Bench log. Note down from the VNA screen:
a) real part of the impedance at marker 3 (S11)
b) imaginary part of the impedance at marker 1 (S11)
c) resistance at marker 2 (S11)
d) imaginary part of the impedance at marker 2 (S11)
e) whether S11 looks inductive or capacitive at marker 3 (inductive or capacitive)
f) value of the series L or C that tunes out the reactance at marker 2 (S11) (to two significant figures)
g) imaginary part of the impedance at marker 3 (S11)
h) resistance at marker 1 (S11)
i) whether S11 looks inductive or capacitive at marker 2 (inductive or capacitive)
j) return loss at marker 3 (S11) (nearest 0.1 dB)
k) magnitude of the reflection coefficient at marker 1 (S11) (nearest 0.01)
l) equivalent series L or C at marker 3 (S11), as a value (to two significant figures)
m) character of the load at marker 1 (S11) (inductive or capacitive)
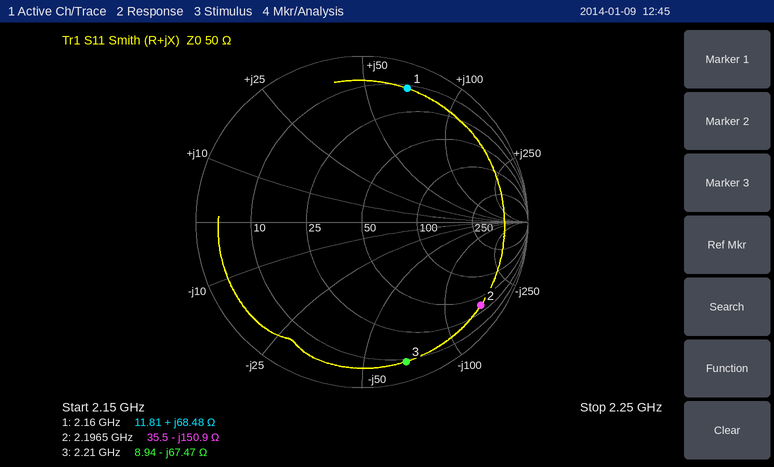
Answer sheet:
8.94 Ω
+68.48 Ω
35.5 Ω
-150.9 Ω
capacitive
11 nH
-67.47 Ω
11.81 Ω
capacitive
1.1 dB
0.85
1.1 pF
inductive
